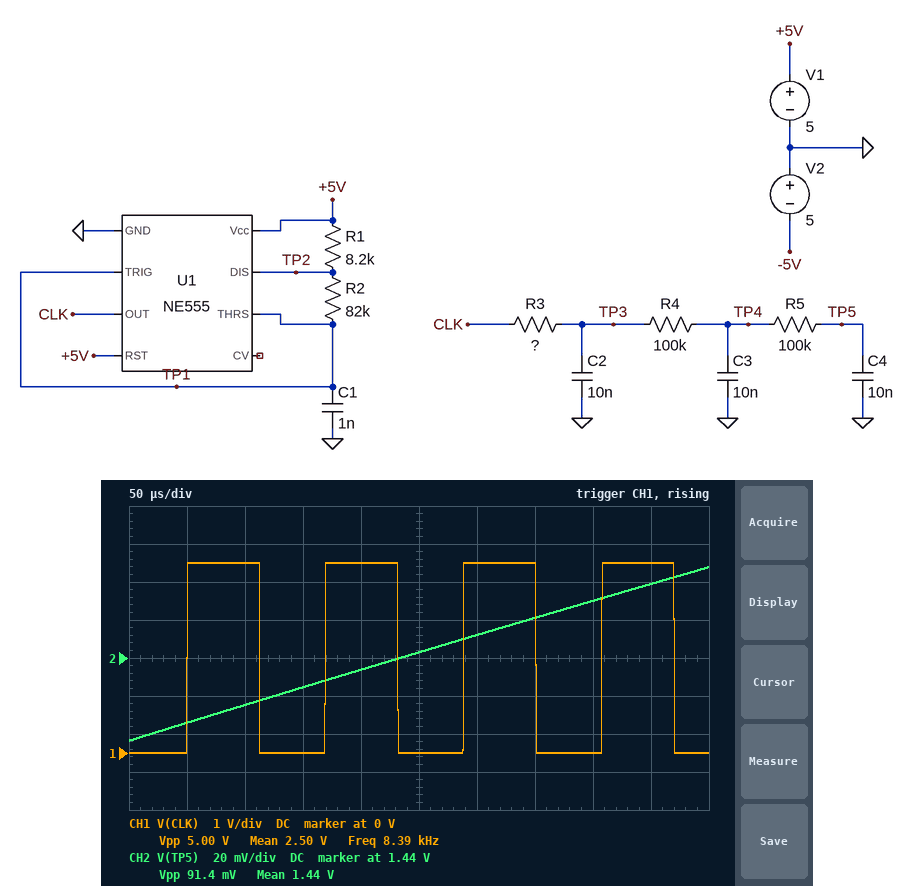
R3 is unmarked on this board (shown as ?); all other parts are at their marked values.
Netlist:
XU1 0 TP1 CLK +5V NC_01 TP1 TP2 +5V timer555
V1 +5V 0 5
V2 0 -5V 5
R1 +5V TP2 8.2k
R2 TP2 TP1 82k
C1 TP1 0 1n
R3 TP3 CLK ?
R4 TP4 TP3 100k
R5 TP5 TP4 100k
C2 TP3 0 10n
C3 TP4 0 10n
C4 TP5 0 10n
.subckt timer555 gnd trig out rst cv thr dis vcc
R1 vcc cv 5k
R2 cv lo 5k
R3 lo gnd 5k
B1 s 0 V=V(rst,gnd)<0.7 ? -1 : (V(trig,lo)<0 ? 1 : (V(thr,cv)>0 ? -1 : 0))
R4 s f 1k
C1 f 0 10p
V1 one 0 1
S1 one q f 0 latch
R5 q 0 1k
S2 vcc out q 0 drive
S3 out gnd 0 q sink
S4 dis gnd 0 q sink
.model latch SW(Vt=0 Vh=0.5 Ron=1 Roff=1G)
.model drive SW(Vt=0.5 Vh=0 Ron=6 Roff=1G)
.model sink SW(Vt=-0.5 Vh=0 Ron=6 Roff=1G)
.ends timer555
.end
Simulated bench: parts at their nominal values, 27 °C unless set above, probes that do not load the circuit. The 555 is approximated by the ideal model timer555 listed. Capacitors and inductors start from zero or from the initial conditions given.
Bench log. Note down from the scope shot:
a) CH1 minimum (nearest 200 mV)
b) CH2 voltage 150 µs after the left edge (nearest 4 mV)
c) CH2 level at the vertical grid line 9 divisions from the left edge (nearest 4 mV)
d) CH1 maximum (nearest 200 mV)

0 V
1.424 V
1.480 V
5.0 V
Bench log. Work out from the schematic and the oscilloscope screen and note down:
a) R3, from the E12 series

150 kΩ
